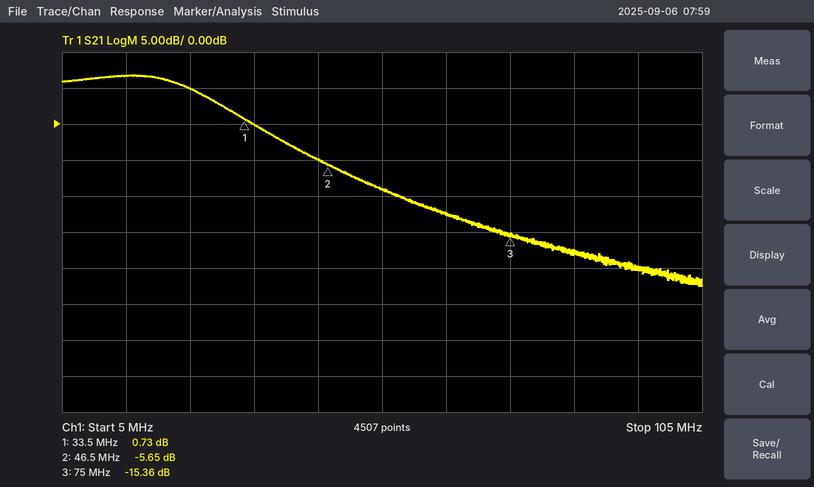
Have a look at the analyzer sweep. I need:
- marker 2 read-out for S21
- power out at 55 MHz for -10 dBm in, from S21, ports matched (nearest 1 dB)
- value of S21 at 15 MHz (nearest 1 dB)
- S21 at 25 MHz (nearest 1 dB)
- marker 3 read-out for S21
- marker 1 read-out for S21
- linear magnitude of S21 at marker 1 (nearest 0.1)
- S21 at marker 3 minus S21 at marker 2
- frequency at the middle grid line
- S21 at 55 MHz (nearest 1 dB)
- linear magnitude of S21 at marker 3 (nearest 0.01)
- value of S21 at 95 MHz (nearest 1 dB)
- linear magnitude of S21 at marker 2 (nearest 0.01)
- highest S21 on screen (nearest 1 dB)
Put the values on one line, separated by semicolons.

-5.65 dB; -19 dBm; 7 dB; 5 dB; -15.36 dB; 0.73 dB; 1.1; -9.71 dB; 55 MHz; -9 dB; 0.17; -20 dB; 0.52; 7 dB
